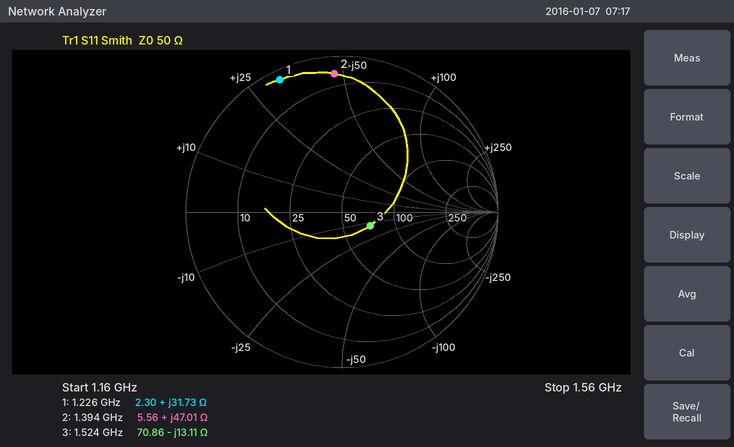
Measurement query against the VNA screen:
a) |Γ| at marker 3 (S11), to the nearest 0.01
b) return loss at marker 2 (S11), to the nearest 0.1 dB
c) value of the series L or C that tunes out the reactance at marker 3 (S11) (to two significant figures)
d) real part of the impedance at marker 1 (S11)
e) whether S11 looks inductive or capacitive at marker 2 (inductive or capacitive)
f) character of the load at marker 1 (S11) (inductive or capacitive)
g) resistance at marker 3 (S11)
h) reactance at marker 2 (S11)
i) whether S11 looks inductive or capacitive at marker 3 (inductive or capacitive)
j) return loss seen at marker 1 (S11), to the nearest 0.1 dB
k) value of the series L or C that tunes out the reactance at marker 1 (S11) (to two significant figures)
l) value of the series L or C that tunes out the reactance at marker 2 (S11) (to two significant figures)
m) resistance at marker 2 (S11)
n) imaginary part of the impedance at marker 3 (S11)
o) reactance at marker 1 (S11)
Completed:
0.20
1.0 dB
1.4 nH
2.30 Ω
inductive
inductive
70.86 Ω
+47.01 Ω
capacitive
0.6 dB
4.1 pF
2.4 pF
5.56 Ω
-13.11 Ω
+31.73 Ω
